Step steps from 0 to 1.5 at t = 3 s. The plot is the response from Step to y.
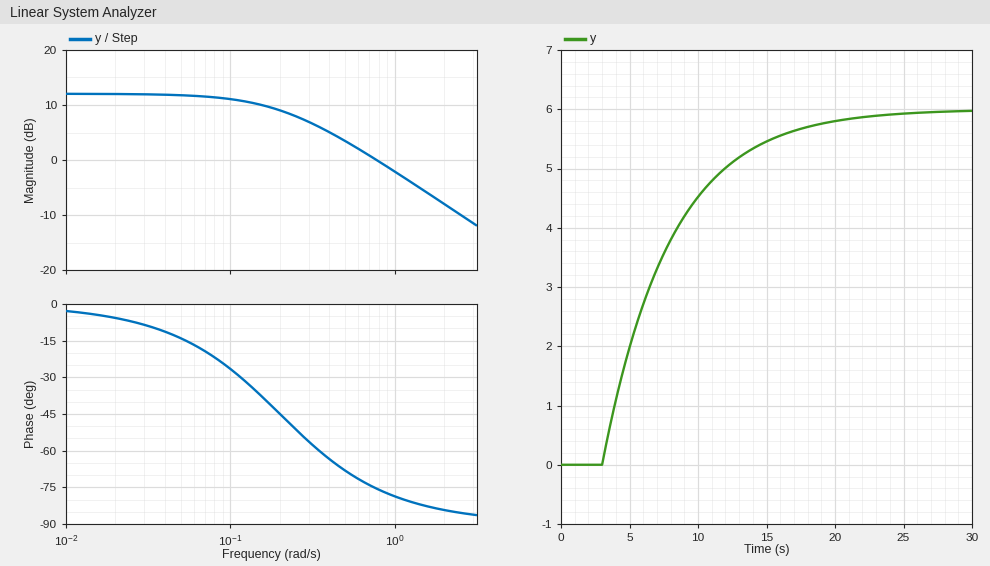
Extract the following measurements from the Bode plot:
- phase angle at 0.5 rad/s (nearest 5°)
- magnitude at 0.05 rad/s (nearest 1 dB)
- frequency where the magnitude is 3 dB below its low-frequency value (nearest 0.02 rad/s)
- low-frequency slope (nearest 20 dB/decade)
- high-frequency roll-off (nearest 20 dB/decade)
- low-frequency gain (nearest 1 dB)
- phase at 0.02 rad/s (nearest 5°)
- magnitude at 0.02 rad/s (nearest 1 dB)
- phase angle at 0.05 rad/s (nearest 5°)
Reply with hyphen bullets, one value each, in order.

- -70°
- 12 dB
- 0.20 rad/s
- 0 dB/decade
- -20 dB/decade
- 12 dB
- -5°
- 12 dB
- -15°
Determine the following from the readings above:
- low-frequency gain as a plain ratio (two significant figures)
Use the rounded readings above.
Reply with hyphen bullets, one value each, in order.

- 4.0
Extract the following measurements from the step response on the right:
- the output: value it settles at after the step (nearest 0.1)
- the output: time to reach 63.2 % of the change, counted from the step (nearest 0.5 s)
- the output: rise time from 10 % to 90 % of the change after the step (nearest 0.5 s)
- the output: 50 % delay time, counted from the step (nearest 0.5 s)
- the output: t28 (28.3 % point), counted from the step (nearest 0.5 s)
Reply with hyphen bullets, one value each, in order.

- 6.0
- 5.0 s
- 11.0 s
- 3.5 s
- 1.5 s
